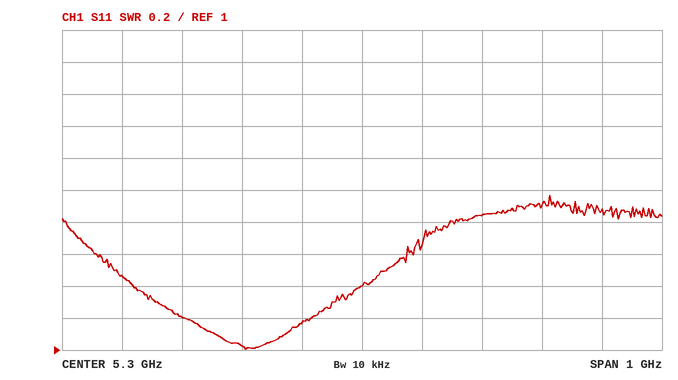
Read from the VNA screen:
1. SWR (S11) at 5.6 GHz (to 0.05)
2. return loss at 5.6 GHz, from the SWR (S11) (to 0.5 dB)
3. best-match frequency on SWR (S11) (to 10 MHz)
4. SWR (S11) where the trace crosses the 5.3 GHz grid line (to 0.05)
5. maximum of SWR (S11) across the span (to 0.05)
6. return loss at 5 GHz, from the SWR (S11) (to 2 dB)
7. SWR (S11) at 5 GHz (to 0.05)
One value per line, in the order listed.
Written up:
1.90
10.0 dB
5.11 GHz
1.40
1.95
20 dB
1.20
